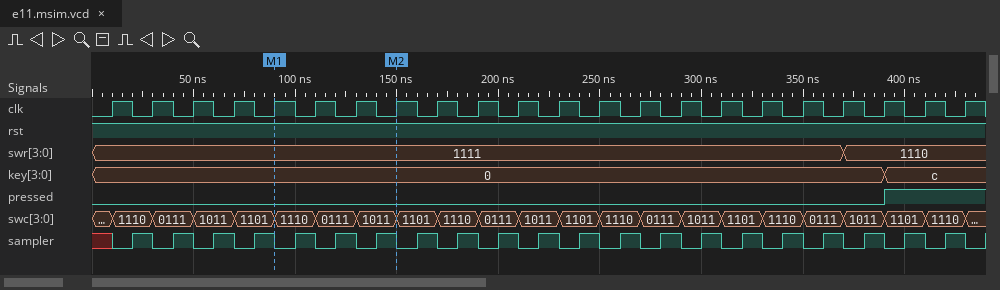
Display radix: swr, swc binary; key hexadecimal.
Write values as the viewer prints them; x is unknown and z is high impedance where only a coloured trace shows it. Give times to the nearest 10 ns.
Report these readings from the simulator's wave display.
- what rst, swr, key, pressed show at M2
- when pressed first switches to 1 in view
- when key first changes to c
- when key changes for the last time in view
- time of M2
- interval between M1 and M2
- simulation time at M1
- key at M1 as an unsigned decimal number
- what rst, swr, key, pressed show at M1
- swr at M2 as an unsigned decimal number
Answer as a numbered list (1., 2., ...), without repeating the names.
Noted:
1. rst=1, swr=1111, key=0, pressed=0
2. 390 ns
3. 390 ns
4. 390 ns
5. 150 ns
6. 60 ns
7. 90 ns
8. 0
9. rst=1, swr=1111, key=0, pressed=0
10. 15
